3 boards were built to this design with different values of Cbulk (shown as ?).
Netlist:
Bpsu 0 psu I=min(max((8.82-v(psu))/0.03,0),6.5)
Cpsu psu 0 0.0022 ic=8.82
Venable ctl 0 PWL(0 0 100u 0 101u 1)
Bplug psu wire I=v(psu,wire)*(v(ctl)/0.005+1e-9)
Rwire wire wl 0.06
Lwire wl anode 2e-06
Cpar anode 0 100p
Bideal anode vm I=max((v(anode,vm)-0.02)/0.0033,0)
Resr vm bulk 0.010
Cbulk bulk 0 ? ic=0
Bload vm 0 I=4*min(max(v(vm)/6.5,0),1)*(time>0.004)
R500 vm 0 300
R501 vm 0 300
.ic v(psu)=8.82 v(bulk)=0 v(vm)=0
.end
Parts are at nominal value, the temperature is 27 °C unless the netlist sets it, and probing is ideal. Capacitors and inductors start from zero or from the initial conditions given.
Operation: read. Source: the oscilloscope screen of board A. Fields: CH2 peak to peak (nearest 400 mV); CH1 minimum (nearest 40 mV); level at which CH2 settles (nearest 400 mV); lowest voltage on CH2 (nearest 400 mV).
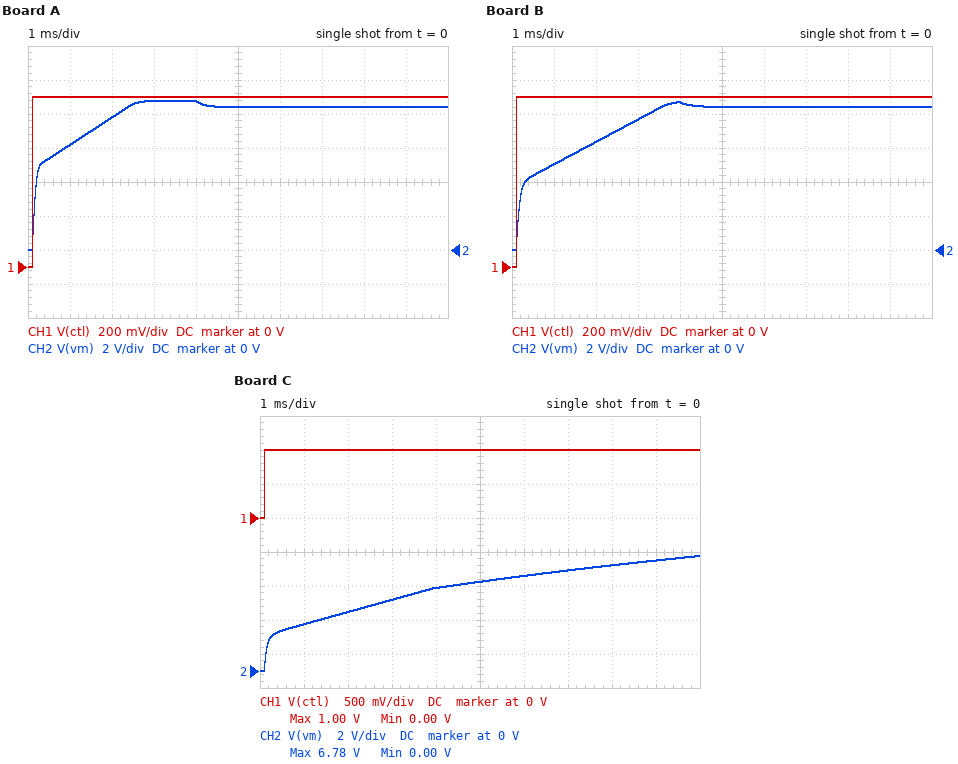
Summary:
8.8 V
0 V
8.4 V
0 V
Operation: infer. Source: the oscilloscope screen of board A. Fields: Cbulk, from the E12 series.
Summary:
1.8 mF
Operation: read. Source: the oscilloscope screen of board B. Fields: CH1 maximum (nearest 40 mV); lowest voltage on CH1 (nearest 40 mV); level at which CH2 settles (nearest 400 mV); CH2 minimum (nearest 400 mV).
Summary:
1.00 V
0 V
8.4 V
0 V
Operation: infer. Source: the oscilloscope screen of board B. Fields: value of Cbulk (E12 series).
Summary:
2.7 mF
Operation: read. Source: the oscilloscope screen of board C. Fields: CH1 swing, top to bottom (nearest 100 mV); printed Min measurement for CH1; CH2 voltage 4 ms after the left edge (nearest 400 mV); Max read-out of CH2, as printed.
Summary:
1.0 V
0.00 V
4.8 V
6.78 V
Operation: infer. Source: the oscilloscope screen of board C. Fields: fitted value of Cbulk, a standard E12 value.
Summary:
6.8 mF
